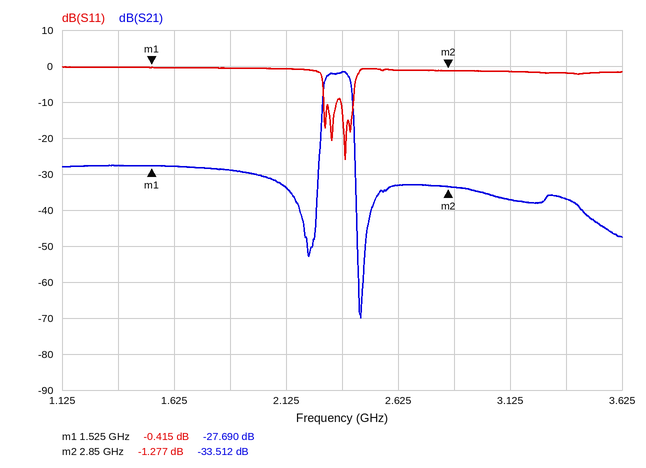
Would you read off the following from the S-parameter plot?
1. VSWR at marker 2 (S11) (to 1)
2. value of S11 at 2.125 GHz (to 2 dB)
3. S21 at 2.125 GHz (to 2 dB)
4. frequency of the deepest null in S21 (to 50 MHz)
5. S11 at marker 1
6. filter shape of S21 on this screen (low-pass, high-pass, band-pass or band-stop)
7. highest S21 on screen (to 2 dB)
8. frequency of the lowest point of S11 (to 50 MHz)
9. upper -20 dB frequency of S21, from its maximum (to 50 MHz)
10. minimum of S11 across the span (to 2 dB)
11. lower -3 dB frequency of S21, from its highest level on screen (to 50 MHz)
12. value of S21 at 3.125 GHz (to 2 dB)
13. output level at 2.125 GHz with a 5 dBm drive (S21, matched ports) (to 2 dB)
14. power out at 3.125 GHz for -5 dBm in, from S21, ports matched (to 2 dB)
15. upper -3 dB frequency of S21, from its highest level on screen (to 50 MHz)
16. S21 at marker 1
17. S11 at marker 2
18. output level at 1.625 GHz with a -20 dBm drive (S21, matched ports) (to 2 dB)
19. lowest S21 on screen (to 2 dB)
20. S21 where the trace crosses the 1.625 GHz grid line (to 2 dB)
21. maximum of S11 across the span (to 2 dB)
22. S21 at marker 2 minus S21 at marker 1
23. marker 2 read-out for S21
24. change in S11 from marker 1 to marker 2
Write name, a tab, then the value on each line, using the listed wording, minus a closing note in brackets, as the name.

VSWR at marker 2 (S11)	14
value of S11 at 2.125 GHz	0 dB
S21 at 2.125 GHz	-34 dB
frequency of the deepest null in S21	2.45 GHz
S11 at marker 1	-0.415 dB
filter shape of S21 on this screen	band-pass
highest S21 on screen	-2 dB
frequency of the lowest point of S11	2.40 GHz
upper -20 dB frequency of S21, from its maximum	2.45 GHz
minimum of S11 across the span	-26 dB
lower -3 dB frequency of S21, from its highest level on screen	2.30 GHz
value of S21 at 3.125 GHz	-38 dB
output level at 2.125 GHz with a 5 dBm drive (S21, matched ports)	-28 dBm
power out at 3.125 GHz for -5 dBm in, from S21, ports matched	-42 dBm
upper -3 dB frequency of S21, from its highest level on screen	2.40 GHz
S21 at marker 1	-27.690 dB
S11 at marker 2	-1.277 dB
output level at 1.625 GHz with a -20 dBm drive (S21, matched ports)	-48 dBm
lowest S21 on screen	-70 dB
S21 where the trace crosses the 1.625 GHz grid line	-28 dB
maximum of S11 across the span	0 dB
S21 at marker 2 minus S21 at marker 1	-5.822 dB
marker 2 read-out for S21	-33.512 dB
change in S11 from marker 1 to marker 2	-0.862 dB
